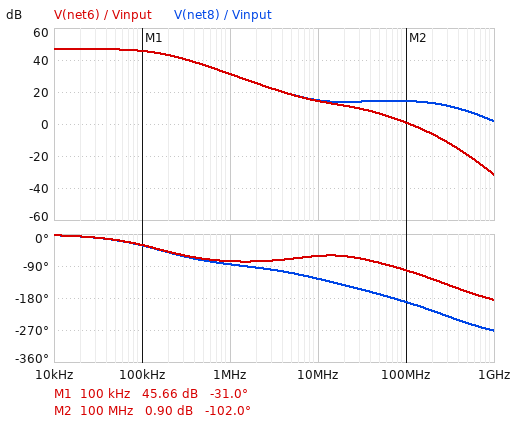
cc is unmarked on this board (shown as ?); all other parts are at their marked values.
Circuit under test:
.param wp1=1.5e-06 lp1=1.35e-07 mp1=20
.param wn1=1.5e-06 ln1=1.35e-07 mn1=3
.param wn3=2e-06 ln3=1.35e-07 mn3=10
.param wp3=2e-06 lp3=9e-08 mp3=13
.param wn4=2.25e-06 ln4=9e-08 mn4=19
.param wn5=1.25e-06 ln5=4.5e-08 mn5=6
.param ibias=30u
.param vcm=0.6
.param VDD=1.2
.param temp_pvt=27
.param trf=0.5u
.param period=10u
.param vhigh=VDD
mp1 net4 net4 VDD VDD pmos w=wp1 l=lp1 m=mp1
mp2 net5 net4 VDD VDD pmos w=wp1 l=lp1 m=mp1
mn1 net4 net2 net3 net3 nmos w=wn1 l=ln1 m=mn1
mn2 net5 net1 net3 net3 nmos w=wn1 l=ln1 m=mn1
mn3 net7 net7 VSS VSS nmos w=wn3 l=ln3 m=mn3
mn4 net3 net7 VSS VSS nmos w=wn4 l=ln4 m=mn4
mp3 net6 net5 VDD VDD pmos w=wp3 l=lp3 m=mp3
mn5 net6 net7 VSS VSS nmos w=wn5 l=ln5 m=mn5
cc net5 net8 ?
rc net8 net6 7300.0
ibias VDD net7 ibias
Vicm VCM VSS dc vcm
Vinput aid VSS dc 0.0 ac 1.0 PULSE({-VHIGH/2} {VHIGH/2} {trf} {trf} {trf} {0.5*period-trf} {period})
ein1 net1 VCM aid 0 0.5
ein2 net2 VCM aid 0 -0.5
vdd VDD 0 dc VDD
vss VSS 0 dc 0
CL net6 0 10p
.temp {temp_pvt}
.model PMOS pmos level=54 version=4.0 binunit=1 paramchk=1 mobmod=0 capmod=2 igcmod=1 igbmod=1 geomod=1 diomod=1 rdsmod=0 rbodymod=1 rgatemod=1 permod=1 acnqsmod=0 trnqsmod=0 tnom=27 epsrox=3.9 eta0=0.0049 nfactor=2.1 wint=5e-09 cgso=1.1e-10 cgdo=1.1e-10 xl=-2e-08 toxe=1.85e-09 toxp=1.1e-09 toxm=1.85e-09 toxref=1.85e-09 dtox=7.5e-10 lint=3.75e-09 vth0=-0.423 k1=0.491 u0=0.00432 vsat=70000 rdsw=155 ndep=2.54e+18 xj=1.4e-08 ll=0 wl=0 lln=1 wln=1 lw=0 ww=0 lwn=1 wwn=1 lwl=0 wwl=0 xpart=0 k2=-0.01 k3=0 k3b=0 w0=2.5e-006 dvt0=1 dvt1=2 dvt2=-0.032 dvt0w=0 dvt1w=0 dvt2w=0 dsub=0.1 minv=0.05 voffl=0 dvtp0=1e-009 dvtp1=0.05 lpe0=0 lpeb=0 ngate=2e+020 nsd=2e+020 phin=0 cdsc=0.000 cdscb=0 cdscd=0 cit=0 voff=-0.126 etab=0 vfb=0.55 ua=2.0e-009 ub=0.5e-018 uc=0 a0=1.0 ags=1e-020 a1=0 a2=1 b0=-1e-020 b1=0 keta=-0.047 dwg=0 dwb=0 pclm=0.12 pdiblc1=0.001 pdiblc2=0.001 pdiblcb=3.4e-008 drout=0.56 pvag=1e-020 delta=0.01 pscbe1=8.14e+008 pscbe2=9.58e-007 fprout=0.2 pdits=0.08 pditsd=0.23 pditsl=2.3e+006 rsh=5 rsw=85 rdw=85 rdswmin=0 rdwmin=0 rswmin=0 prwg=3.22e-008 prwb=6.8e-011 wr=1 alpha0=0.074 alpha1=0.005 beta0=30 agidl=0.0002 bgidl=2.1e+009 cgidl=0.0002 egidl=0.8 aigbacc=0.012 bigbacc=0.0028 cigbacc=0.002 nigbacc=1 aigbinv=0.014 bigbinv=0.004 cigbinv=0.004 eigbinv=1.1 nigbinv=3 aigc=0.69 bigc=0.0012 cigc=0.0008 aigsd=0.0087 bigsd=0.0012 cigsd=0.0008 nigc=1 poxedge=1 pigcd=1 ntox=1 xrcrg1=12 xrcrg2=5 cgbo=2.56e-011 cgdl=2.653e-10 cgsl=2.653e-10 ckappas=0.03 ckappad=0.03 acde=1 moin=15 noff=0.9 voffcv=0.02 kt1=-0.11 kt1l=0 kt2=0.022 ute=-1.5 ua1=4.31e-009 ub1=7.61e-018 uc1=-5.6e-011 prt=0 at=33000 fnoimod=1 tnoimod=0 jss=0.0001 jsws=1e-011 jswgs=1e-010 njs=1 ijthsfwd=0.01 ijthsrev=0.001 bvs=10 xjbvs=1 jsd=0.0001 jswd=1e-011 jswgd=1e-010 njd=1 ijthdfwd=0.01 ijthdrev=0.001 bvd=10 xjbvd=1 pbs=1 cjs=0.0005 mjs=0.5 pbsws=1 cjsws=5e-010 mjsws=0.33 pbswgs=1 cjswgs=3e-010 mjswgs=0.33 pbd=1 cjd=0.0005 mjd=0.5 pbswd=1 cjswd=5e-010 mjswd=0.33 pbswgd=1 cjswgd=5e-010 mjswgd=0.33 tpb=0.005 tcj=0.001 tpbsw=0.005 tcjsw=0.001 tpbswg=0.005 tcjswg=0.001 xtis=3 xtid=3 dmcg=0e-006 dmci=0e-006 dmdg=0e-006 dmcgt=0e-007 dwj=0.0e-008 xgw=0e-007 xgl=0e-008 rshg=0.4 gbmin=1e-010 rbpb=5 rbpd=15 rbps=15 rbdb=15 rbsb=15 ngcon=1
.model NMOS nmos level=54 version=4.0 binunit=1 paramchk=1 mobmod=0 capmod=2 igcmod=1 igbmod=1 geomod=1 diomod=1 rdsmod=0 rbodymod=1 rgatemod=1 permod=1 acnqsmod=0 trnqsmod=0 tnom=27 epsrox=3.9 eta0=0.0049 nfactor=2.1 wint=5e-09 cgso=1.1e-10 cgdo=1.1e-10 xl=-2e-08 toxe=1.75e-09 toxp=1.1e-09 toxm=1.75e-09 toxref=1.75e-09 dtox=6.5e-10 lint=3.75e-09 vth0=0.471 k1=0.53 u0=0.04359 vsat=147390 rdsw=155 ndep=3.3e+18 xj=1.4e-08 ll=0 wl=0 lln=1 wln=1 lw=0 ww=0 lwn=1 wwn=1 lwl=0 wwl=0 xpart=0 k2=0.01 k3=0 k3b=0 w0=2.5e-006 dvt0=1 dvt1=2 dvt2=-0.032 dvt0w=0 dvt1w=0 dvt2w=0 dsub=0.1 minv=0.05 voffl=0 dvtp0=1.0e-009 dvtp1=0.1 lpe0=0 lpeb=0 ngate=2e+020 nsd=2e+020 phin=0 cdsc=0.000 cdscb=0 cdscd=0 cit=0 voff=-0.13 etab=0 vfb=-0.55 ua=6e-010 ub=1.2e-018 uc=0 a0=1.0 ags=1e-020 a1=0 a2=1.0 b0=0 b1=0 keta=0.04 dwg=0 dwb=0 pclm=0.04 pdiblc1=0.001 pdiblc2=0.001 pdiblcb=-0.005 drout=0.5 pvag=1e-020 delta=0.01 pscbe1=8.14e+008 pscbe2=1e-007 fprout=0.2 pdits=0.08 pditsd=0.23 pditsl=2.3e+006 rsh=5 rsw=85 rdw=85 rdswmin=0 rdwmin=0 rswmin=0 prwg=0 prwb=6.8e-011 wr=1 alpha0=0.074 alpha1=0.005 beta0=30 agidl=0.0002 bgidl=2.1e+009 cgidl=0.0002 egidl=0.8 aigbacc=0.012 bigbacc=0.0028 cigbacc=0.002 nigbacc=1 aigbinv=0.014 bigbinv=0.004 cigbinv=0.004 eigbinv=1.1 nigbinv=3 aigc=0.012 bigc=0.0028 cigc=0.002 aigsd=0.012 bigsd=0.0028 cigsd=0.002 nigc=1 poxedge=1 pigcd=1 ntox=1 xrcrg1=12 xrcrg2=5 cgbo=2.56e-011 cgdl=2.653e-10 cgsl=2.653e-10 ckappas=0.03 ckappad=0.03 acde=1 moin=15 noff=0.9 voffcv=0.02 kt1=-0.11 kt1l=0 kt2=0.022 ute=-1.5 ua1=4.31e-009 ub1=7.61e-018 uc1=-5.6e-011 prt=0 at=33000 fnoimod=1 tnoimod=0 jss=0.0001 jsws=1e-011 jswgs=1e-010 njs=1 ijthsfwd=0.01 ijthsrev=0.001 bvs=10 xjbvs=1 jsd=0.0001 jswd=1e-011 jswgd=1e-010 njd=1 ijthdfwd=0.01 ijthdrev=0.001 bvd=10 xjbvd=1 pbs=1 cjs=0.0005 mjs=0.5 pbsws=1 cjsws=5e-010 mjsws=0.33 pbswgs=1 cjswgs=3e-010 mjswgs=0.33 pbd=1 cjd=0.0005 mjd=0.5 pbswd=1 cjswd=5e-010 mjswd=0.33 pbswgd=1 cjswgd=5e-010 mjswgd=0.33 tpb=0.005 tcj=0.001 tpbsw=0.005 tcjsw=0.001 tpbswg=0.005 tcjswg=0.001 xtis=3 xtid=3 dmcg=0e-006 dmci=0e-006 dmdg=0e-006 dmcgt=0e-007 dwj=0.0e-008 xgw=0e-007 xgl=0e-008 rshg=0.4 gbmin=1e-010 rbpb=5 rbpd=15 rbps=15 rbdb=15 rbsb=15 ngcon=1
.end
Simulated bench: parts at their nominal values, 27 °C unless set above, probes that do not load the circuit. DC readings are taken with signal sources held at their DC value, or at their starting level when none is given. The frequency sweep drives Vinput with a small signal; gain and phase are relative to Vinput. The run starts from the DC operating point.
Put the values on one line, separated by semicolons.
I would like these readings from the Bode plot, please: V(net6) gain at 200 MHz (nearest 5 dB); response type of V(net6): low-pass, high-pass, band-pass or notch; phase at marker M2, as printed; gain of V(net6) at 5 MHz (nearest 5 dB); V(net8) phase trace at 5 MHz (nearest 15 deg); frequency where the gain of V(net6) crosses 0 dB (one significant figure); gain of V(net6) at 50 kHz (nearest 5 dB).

-5 dB; low-pass; -102.0 deg; 20 dB; -105 deg; 100 MHz; 45 dB
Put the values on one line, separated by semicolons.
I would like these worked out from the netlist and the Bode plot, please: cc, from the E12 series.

2.7 pF
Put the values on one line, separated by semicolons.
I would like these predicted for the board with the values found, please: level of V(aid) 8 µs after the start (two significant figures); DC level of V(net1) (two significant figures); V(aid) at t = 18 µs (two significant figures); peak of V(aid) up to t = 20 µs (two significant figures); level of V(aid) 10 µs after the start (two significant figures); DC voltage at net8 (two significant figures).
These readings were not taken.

-600 mV; 600 mV; -600 mV; 600 mV; -600 mV; 150 mV
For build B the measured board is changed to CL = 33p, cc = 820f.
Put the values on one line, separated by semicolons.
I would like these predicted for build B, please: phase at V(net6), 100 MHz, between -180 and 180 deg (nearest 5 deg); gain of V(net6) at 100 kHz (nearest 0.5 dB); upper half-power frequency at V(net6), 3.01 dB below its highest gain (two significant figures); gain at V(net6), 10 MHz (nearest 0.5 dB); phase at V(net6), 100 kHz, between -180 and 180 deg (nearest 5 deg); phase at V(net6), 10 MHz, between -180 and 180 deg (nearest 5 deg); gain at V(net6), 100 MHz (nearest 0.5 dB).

-120 deg; 47.0 dB; 440 kHz; 17.5 dB; -15 deg; -115 deg; -9.5 dB
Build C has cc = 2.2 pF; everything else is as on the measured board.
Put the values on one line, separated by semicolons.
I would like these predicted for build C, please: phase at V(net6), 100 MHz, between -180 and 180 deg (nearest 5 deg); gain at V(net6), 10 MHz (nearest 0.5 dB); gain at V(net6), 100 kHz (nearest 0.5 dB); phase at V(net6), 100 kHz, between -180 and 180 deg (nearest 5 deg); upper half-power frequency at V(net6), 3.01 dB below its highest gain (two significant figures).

-105 deg; 15.0 dB; 46.0 dB; -25 deg; 200 kHz
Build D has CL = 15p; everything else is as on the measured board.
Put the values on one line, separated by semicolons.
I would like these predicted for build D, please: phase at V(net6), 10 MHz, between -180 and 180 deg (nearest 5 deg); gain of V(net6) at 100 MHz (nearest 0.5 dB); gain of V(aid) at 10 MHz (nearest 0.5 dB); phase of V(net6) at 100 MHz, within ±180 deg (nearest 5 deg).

-70 deg; -2.5 dB; 0 dB; -105 deg
